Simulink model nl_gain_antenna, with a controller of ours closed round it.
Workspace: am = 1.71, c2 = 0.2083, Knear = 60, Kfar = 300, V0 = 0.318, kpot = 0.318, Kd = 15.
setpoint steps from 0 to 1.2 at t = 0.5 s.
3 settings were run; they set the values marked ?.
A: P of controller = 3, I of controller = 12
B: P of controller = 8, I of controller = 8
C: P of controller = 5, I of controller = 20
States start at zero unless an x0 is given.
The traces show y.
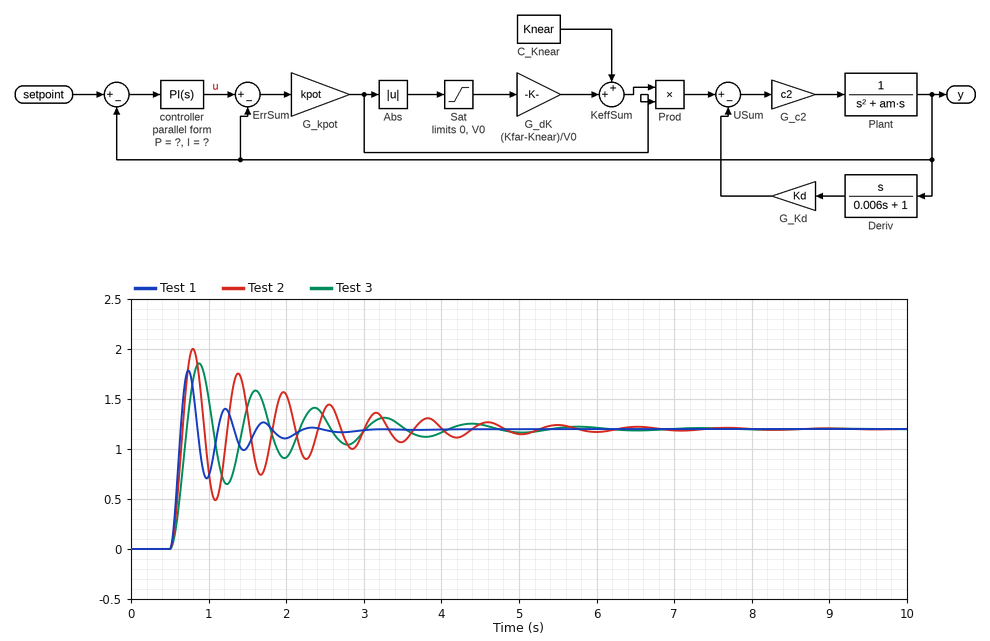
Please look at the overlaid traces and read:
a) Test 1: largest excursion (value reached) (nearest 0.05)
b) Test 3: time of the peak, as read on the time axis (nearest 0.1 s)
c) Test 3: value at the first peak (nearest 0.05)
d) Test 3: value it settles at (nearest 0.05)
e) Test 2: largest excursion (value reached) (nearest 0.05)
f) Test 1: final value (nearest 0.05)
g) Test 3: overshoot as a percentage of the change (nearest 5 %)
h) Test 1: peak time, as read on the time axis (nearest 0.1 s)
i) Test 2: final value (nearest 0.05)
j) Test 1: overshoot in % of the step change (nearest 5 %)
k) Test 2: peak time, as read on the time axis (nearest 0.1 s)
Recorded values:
1.80
0.9 s
1.85
1.20
2.00
1.20
55 %
0.7 s
1.20
50 %
0.8 s
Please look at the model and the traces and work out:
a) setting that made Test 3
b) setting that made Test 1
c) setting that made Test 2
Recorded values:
A
B
C
